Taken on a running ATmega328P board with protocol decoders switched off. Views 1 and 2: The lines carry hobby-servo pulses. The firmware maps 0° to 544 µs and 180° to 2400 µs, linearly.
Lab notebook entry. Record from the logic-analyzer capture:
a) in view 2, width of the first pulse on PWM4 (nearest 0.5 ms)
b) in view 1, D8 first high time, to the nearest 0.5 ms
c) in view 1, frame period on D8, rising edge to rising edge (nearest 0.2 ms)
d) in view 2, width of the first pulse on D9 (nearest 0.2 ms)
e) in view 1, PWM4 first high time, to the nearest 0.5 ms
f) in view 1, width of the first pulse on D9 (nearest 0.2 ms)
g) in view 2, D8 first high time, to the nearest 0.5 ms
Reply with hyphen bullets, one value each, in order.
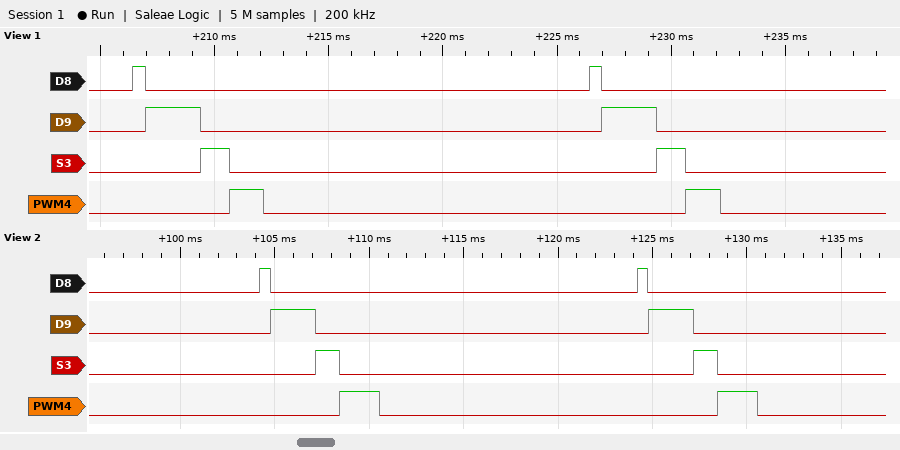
- 2.0 ms
- 0.5 ms
- 20.0 ms
- 2.4 ms
- 1.5 ms
- 2.4 ms
- 0.5 ms
